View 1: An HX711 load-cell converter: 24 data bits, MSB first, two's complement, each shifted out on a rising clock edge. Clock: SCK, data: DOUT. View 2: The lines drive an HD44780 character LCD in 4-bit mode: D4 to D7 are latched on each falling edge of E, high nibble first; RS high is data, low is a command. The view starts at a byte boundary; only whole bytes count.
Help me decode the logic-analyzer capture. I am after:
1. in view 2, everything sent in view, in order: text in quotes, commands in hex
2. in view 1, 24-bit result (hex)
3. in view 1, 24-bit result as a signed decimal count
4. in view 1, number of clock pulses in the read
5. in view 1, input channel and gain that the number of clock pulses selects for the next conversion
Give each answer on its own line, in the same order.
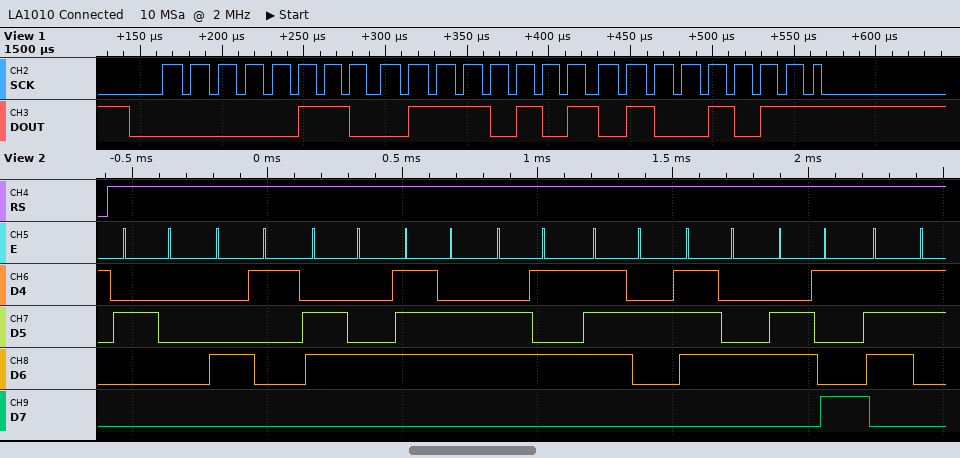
" Advertis"
0x06754B
423243
25
channel A, gain 128
